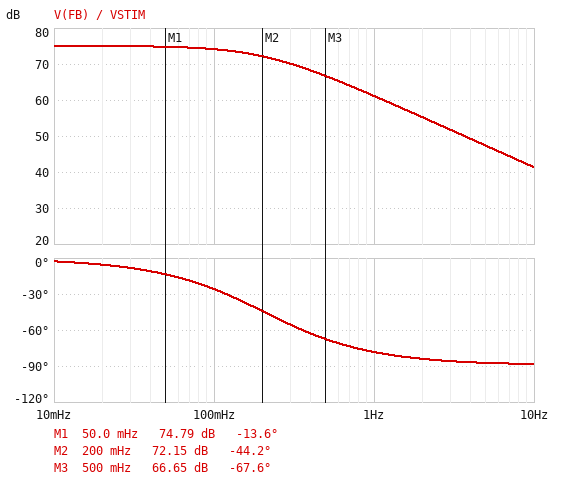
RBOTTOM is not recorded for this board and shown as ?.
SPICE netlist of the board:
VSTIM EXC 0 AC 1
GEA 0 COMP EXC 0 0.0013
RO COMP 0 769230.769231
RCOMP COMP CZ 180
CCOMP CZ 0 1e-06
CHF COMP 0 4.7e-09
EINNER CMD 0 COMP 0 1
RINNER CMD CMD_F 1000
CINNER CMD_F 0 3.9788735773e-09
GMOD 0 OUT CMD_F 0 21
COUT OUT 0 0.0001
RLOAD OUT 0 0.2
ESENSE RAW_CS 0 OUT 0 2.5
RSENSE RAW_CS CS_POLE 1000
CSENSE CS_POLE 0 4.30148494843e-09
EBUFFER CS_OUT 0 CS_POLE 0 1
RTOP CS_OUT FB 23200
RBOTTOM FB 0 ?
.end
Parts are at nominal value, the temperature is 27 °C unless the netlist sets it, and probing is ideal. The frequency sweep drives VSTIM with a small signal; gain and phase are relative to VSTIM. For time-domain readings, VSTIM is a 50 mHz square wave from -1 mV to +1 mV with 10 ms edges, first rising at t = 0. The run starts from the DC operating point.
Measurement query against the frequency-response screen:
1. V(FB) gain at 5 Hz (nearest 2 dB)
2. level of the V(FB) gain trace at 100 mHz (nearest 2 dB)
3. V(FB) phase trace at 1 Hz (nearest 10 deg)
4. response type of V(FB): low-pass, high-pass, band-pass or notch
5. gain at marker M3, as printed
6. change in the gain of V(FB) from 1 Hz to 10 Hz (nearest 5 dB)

48 dB
74 dB
-80 deg
low-pass
66.65 dB
-20 dB
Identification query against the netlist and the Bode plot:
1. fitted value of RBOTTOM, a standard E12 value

27 kΩ
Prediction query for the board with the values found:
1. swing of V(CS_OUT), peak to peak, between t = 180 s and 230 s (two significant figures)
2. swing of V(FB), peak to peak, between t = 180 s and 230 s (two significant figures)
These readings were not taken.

21 V
11 V
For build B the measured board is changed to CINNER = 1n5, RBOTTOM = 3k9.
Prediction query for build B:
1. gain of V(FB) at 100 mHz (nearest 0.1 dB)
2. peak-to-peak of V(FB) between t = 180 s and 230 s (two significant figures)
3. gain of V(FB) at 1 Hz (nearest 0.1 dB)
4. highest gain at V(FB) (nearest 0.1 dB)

62.7 dB
3.0 V
49.7 dB
63.6 dB
